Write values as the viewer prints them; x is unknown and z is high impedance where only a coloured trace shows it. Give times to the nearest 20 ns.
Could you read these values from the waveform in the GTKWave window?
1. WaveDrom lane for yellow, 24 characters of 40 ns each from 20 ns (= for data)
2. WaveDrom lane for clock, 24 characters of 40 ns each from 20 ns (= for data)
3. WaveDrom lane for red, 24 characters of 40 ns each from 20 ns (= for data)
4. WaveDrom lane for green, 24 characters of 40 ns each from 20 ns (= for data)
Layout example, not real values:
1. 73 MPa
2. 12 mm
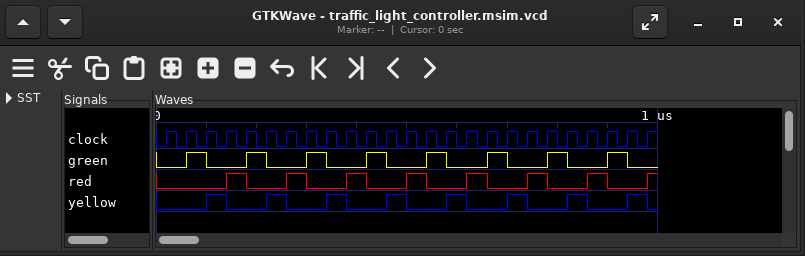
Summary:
1. {name: 'yellow', wave: '0.10.10.10.10.10.10.10.1'}
2. {name: 'clock', wave: 'p.......................'}
3. {name: 'red', wave: '0..10.10.10.10.10.10.10.'}
4. {name: 'green', wave: '010.10.10.10.10.10.10.10'}
